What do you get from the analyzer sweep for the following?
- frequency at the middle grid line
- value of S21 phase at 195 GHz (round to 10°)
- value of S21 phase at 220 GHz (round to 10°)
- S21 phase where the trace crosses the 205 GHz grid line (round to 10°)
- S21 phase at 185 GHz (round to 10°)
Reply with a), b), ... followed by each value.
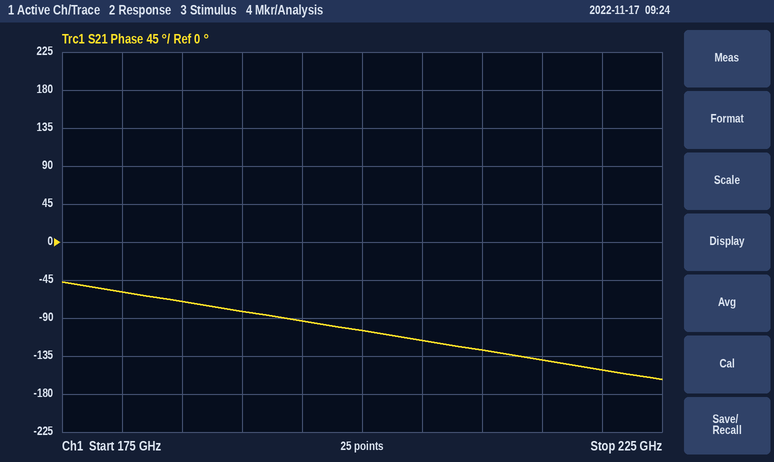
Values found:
a) 200 GHz
b) -90°
c) -150°
d) -120°
e) -70°
